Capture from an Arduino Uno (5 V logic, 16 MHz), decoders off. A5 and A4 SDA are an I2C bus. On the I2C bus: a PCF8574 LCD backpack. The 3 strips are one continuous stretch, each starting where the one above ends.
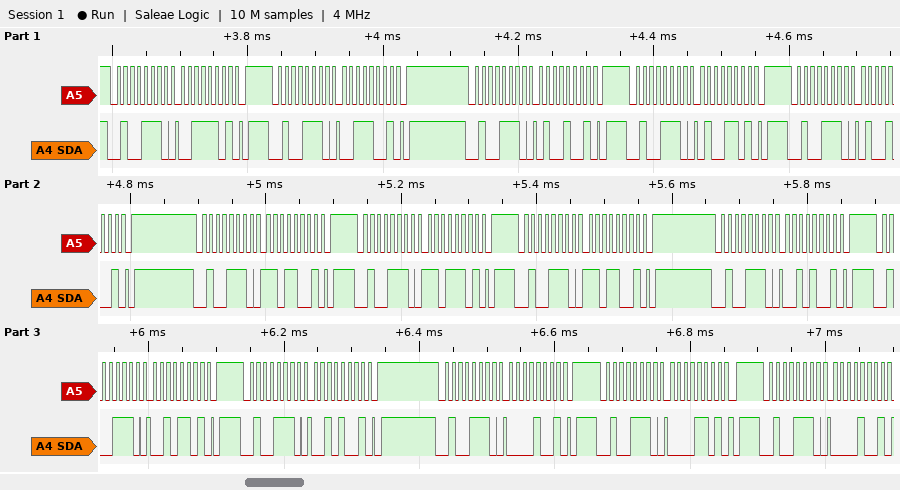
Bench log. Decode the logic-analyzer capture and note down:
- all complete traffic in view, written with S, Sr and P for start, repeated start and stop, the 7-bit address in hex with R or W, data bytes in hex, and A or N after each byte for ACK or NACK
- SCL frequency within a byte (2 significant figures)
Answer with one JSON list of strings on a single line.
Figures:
["S 27W A 3D A P S 27W A 39 A P S 27W A 49 A P S 27W A 4D A P S 27W A 49 A P S 27W A D9 A P S 27W A DD A P S 27W A D9 A P S 27W A 29 A P S 27W A 2D A P S 27W A 29 A P S 27W A 09 A P S 27W A 0D A P S 27W A 09 A", "100 kHz"]
